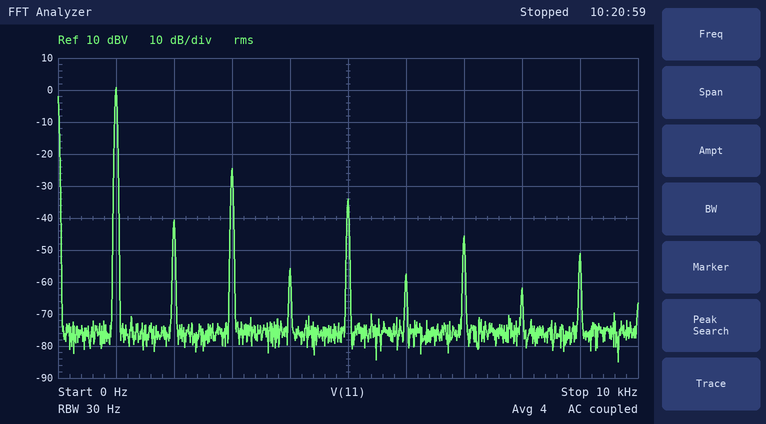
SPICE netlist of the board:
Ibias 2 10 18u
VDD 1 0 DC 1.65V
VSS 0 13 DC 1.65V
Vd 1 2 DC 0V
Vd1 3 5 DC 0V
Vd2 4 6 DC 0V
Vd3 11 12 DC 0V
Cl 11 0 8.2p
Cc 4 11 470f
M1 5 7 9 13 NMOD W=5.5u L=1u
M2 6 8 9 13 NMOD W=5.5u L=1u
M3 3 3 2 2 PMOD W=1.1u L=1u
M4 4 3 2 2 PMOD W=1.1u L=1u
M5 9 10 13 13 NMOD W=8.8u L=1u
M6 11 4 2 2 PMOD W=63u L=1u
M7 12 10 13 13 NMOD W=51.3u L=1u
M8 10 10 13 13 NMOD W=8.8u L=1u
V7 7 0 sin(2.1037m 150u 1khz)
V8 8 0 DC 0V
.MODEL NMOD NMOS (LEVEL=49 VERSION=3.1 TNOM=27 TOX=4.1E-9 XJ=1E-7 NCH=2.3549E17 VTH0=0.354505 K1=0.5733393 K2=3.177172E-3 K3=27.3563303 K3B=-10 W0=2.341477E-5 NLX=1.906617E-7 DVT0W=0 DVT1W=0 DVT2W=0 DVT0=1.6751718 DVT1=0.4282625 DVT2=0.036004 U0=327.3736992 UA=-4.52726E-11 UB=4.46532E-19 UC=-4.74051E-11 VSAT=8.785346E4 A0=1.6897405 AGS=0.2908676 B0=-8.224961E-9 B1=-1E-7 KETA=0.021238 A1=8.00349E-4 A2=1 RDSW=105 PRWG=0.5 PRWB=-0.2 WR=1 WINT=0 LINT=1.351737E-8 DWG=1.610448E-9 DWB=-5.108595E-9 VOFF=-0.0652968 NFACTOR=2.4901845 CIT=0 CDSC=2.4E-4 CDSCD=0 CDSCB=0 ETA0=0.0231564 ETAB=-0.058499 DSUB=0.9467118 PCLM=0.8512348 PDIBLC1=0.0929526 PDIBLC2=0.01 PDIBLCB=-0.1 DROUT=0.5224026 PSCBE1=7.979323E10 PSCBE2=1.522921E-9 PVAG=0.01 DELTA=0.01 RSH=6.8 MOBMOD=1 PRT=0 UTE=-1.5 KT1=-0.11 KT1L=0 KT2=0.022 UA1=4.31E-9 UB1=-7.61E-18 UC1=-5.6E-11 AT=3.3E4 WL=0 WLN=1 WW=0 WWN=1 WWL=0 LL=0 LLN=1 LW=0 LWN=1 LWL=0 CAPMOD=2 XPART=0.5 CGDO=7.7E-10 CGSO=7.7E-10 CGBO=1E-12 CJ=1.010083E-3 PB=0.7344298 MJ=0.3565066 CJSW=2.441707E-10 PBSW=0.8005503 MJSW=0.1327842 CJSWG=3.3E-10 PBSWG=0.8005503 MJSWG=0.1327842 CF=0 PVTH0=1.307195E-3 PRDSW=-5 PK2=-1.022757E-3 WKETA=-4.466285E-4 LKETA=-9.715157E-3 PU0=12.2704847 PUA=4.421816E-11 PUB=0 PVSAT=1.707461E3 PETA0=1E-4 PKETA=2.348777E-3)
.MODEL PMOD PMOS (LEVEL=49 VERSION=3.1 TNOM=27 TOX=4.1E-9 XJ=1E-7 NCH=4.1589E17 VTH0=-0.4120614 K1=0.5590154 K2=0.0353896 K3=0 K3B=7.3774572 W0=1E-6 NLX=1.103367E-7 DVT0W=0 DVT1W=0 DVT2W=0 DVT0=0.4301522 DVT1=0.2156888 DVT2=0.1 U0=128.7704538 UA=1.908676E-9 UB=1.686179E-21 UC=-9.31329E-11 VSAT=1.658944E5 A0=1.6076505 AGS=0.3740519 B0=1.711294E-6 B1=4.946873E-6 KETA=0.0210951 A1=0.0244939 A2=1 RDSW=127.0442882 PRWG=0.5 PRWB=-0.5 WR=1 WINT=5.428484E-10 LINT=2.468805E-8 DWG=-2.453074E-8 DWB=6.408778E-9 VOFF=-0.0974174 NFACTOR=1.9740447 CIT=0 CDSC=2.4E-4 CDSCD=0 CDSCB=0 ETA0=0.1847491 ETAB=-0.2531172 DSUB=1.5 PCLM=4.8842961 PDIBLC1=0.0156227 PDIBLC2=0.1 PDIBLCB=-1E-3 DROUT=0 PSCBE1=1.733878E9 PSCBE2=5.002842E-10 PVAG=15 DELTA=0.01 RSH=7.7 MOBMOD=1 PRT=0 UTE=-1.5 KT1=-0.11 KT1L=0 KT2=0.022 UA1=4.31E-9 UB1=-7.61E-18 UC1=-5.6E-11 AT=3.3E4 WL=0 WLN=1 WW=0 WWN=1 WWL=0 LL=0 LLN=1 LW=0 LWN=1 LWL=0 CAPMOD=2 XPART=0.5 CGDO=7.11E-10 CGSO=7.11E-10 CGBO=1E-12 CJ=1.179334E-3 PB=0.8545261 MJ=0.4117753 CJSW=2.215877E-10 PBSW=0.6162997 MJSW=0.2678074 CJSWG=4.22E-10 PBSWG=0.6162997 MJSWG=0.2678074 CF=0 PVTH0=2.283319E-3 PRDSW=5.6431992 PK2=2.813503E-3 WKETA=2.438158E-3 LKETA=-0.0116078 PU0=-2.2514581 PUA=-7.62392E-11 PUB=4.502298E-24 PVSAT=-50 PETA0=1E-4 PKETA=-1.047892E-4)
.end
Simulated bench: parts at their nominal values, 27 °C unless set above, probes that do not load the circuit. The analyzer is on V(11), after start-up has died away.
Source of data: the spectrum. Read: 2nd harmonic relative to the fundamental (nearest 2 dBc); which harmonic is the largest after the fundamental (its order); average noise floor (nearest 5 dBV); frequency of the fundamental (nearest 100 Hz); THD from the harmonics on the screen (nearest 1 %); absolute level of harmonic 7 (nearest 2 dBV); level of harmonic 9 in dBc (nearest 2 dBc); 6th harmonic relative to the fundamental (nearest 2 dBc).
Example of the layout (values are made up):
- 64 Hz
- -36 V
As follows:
- -42 dBc
- 3
- -75 dBV
- 1.0 kHz
- 6 %
- -46 dBV
- -52 dBc
- -58 dBc
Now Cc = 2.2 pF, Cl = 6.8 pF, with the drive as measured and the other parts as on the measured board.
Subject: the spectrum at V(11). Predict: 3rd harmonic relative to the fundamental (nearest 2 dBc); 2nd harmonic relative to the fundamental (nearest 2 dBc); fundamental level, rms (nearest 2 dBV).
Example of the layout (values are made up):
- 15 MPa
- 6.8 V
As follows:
- -58 dBc
- -60 dBc
- -2 dBV
